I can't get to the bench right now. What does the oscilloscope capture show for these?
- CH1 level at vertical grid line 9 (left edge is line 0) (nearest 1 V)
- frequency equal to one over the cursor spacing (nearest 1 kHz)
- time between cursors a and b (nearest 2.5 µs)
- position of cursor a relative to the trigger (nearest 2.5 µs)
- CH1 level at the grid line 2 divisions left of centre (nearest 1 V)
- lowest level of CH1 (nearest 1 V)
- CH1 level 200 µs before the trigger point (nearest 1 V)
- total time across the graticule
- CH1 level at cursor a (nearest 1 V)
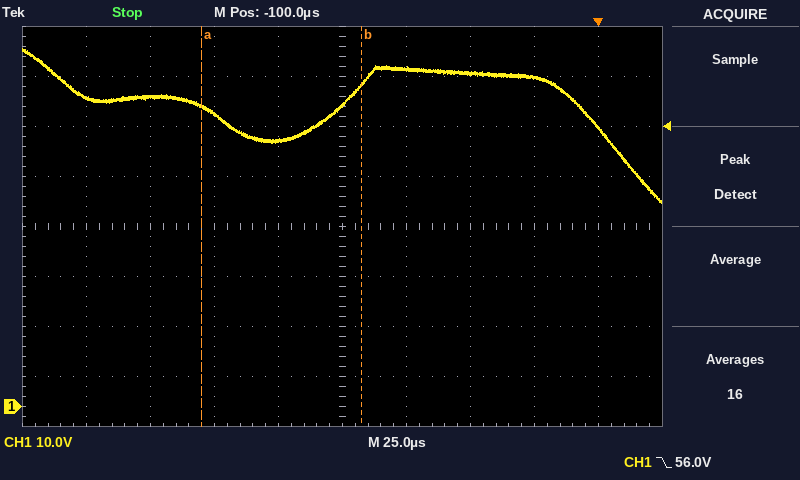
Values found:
56 V
16 kHz
62.5 µs
-155.0 µs
59 V
41 V
62 V
250 µs
60 V
